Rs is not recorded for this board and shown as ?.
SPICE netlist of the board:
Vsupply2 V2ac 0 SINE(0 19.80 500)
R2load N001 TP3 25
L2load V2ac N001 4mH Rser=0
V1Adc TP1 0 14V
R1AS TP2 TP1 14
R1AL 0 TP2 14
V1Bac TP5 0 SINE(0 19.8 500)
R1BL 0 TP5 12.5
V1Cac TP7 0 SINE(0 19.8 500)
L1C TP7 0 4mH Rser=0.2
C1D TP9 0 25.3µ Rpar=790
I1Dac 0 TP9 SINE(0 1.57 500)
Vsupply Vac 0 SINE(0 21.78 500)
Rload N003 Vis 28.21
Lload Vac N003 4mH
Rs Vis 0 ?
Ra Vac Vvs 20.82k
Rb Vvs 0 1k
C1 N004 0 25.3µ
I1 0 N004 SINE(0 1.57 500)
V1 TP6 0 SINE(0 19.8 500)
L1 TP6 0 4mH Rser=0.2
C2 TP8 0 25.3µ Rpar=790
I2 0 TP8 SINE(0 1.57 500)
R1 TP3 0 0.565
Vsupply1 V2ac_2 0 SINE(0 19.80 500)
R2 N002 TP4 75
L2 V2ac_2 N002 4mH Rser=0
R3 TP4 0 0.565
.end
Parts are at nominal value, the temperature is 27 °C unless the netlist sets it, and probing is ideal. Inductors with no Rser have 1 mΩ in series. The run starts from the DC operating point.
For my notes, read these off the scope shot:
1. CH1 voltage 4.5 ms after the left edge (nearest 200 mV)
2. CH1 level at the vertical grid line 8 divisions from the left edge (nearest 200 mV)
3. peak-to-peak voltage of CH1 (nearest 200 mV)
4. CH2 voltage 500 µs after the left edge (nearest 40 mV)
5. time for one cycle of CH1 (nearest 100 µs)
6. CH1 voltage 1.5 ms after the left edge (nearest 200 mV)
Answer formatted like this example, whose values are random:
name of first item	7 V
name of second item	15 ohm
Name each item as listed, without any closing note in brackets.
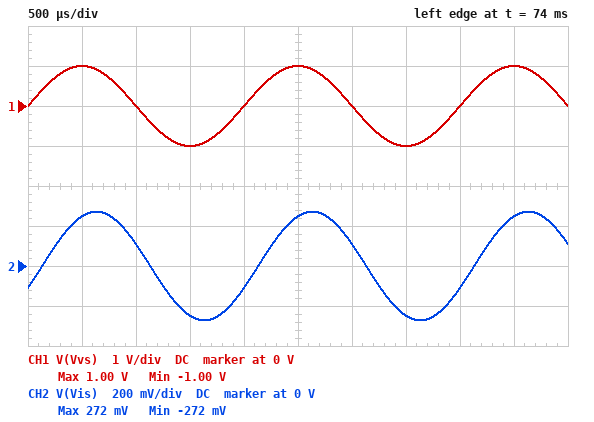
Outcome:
CH1 voltage 4.5 ms after the left edge	1.0 V
CH1 level at the vertical grid line 8 divisions from the left edge	0 V
peak-to-peak voltage of CH1	2.0 V
CH2 voltage 500 µs after the left edge	240 mV
time for one cycle of CH1	2.0 ms
CH1 voltage 1.5 ms after the left edge	-1.0 V
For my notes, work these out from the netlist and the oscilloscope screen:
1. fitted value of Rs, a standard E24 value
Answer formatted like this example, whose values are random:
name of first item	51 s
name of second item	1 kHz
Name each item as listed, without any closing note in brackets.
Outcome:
fitted value of Rs, a standard E24 value	0.39 Ω
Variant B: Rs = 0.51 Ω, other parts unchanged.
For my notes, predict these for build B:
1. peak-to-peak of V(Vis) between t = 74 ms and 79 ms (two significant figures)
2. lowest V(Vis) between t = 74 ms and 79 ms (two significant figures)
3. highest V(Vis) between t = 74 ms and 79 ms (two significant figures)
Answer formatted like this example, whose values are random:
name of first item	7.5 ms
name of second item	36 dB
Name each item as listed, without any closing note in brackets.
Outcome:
peak-to-peak of V(Vis) between t = 74 ms and 79 ms	710 mV
lowest V(Vis) between t = 74 ms and 79 ms	-350 mV
highest V(Vis) between t = 74 ms and 79 ms	350 mV
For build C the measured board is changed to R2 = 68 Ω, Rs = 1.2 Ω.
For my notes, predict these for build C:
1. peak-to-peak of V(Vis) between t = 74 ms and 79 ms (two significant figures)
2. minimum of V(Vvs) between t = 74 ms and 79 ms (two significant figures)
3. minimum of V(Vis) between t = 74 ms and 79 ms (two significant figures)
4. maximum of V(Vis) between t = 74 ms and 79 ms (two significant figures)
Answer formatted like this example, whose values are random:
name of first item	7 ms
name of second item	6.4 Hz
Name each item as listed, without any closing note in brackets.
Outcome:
peak-to-peak of V(Vis) between t = 74 ms and 79 ms	1.6 V
minimum of V(Vvs) between t = 74 ms and 79 ms	-1.0 V
minimum of V(Vis) between t = 74 ms and 79 ms	-820 mV
maximum of V(Vis) between t = 74 ms and 79 ms	820 mV
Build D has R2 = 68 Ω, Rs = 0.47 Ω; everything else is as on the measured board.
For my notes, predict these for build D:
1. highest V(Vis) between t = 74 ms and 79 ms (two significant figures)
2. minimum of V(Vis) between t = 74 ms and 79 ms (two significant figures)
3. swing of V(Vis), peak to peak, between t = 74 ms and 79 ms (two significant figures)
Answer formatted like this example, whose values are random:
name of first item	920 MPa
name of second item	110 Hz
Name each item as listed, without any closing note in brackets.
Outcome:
highest V(Vis) between t = 74 ms and 79 ms	330 mV
minimum of V(Vis) between t = 74 ms and 79 ms	-330 mV
swing of V(Vis), peak to peak, between t = 74 ms and 79 ms	650 mV
